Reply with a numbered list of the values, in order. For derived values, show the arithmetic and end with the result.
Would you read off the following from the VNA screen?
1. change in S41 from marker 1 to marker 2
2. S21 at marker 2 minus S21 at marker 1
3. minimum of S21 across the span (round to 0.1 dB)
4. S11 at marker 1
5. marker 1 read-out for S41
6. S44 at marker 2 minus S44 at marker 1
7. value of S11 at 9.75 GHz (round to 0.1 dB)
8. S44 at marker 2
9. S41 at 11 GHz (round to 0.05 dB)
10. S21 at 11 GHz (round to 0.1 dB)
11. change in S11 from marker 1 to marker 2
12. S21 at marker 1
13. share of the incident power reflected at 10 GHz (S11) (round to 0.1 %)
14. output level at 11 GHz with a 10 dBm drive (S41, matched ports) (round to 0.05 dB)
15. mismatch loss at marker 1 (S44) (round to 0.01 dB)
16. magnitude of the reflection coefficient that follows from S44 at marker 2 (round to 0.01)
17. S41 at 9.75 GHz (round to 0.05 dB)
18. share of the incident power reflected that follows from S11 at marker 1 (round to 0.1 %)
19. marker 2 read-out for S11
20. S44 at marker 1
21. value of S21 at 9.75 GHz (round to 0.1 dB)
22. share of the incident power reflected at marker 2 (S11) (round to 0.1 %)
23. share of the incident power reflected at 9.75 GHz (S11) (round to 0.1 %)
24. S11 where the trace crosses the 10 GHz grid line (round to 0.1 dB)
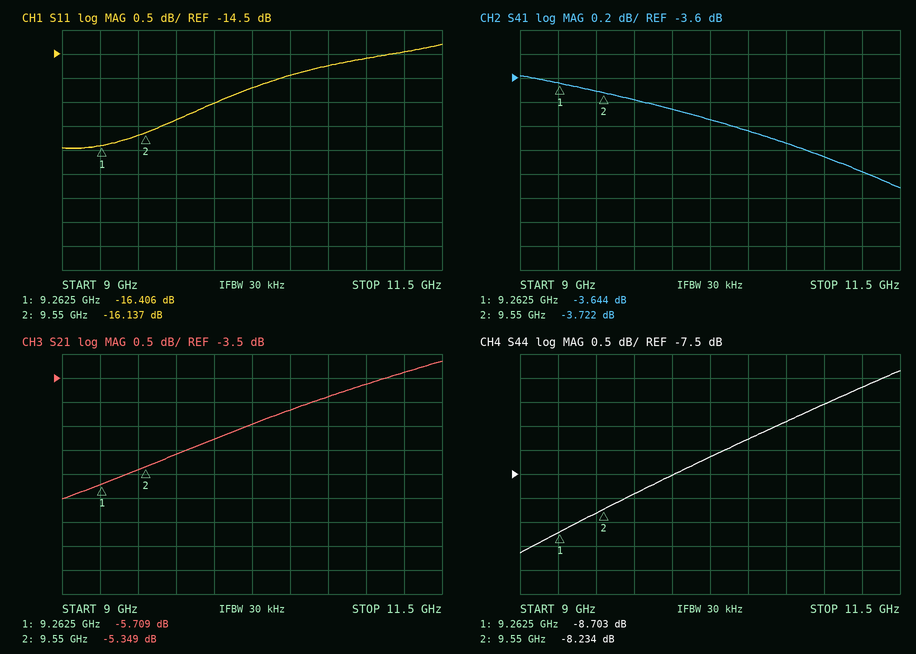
1. -3.722 − (-3.644) = -0.078 dB
2. -5.349 − (-5.709) = 0.360 dB
3. -6.0 dB
4. -16.406 dB
5. -3.644 dB
6. -8.234 − (-8.703) = 0.469 dB
7. -15.9 dB
8. -8.234 dB
9. -4.25 dB
10. -3.6 dB
11. -16.137 − (-16.406) = 0.269 dB
12. -5.709 dB
13. 10^(-15.5/10) ≈ 2.8 %
14. 10 dBm + (-4.25 dB) = 5.75 dBm
15. −10 log10(1 − 10^(-8.703/10)) ≈ 0.63 dB
16. 10^(-8.234/20) ≈ 0.39
17. -3.80 dB
18. 10^(-16.406/10) ≈ 2.3 %
19. -16.137 dB
20. -8.703 dB
21. -5.1 dB
22. 10^(-16.137/10) ≈ 2.4 %
23. 10^(-15.9/10) ≈ 2.6 %
24. -15.5 dB
